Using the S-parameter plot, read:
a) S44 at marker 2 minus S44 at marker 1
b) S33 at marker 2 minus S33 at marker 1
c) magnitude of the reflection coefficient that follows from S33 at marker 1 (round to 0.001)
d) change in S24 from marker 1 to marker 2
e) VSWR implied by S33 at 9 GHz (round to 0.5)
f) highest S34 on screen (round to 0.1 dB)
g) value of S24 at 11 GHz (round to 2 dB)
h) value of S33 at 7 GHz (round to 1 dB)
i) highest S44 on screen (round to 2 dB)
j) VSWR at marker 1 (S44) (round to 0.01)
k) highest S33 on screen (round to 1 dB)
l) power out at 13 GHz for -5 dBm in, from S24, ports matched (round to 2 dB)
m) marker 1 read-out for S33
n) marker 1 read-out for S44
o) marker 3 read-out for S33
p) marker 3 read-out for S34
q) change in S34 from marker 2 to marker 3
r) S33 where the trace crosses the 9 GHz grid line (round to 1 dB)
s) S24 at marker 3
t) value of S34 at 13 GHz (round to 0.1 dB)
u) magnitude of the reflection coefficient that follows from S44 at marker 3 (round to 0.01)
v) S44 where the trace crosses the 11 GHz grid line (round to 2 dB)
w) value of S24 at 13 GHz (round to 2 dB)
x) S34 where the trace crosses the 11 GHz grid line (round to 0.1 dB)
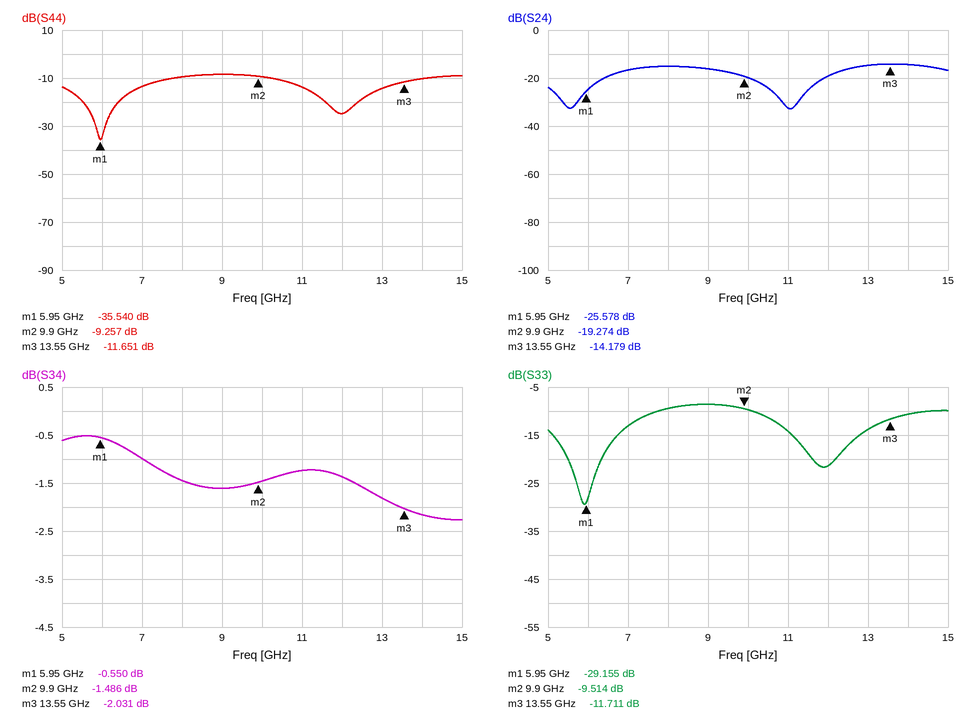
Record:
26.283 dB
19.641 dB
0.035
6.304 dB
2.0
-0.5 dB
-32 dB
-13 dB
-8 dB
1.03
-9 dB
-20 dBm
-29.155 dB
-35.540 dB
-11.711 dB
-2.031 dB
-0.545 dB
-9 dB
-14.179 dB
-1.8 dB
0.26
-14 dB
-14 dB
-1.2 dB
